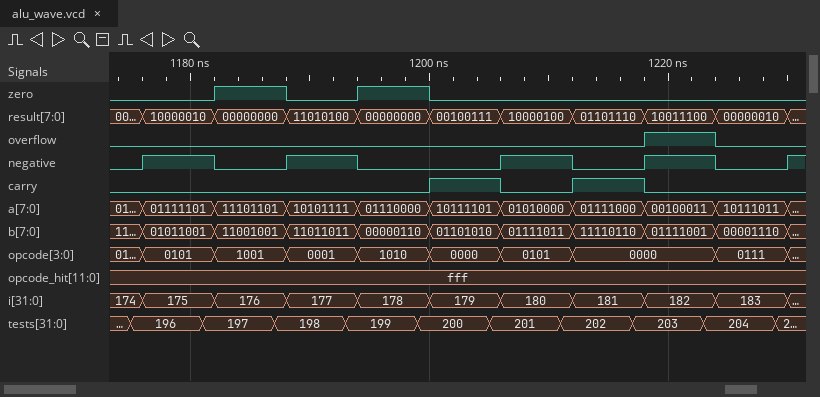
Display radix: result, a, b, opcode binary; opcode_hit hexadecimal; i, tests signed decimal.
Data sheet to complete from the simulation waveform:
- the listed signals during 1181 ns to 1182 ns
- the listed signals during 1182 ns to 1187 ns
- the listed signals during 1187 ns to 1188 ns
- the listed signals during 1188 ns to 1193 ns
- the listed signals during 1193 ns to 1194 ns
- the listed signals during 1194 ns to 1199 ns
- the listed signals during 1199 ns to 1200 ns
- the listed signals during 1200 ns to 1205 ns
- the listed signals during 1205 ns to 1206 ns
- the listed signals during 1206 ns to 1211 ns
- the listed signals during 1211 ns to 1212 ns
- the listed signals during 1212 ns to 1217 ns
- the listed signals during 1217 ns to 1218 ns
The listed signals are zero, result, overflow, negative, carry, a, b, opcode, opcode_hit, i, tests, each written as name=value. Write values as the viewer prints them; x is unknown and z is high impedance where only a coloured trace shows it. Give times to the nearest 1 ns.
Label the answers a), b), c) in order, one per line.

a) zero=0, result=10000010, overflow=0, negative=1, carry=0, a=01111101, b=01011001, opcode=0101, opcode_hit=fff, i=175, tests=197
b) zero=1, result=00000000, overflow=0, negative=0, carry=0, a=11101101, b=11001001, opcode=1001, opcode_hit=fff, i=176, tests=197
c) zero=1, result=00000000, overflow=0, negative=0, carry=0, a=11101101, b=11001001, opcode=1001, opcode_hit=fff, i=176, tests=198
d) zero=0, result=11010100, overflow=0, negative=1, carry=0, a=10101111, b=11011011, opcode=0001, opcode_hit=fff, i=177, tests=198
e) zero=0, result=11010100, overflow=0, negative=1, carry=0, a=10101111, b=11011011, opcode=0001, opcode_hit=fff, i=177, tests=199
f) zero=1, result=00000000, overflow=0, negative=0, carry=0, a=01110000, b=00000110, opcode=1010, opcode_hit=fff, i=178, tests=199
g) zero=1, result=00000000, overflow=0, negative=0, carry=0, a=01110000, b=00000110, opcode=1010, opcode_hit=fff, i=178, tests=200
h) zero=0, result=00100111, overflow=0, negative=0, carry=1, a=10111101, b=01101010, opcode=0000, opcode_hit=fff, i=179, tests=200
i) zero=0, result=00100111, overflow=0, negative=0, carry=1, a=10111101, b=01101010, opcode=0000, opcode_hit=fff, i=179, tests=201
j) zero=0, result=10000100, overflow=0, negative=1, carry=0, a=01010000, b=01111011, opcode=0101, opcode_hit=fff, i=180, tests=201
k) zero=0, result=10000100, overflow=0, negative=1, carry=0, a=01010000, b=01111011, opcode=0101, opcode_hit=fff, i=180, tests=202
l) zero=0, result=01101110, overflow=0, negative=0, carry=1, a=01111000, b=11110110, opcode=0000, opcode_hit=fff, i=181, tests=202
m) zero=0, result=01101110, overflow=0, negative=0, carry=1, a=01111000, b=11110110, opcode=0000, opcode_hit=fff, i=181, tests=203
